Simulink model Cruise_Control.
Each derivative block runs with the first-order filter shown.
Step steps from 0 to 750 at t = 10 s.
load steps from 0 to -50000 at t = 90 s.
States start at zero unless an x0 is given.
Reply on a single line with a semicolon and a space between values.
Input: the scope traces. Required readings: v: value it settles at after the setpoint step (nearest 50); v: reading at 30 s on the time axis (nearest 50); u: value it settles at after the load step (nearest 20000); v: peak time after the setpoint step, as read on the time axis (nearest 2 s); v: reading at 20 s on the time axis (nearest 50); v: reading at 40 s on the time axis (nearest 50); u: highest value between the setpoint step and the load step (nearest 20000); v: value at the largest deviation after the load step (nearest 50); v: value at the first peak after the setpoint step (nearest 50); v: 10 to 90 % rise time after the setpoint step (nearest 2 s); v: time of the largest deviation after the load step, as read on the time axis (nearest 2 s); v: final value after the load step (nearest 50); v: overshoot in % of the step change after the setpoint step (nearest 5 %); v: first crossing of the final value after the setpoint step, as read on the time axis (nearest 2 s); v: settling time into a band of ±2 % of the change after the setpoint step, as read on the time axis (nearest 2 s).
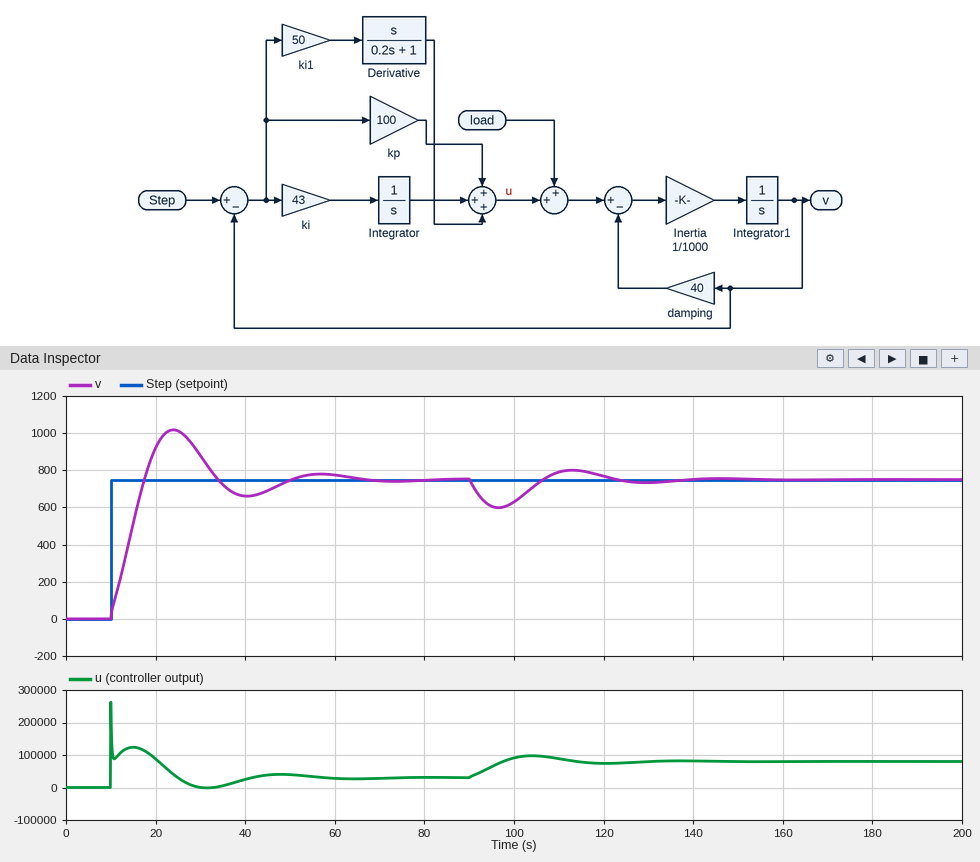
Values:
750; 900; 80000; 24 s; 900; 650; 260000; 600; 1000; 6 s; 96 s; 750; 35 %; 18 s; 62 s
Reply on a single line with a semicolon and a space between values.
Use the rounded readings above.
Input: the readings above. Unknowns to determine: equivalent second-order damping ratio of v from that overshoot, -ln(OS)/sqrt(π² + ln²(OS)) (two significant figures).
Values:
0.32
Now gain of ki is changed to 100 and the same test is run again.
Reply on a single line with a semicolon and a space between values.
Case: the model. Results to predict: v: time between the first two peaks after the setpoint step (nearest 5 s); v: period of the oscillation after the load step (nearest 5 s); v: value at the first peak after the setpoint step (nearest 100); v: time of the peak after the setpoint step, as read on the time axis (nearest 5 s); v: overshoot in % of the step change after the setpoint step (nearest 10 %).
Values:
20 s; 20 s; 1100; 20 s; 50 %
